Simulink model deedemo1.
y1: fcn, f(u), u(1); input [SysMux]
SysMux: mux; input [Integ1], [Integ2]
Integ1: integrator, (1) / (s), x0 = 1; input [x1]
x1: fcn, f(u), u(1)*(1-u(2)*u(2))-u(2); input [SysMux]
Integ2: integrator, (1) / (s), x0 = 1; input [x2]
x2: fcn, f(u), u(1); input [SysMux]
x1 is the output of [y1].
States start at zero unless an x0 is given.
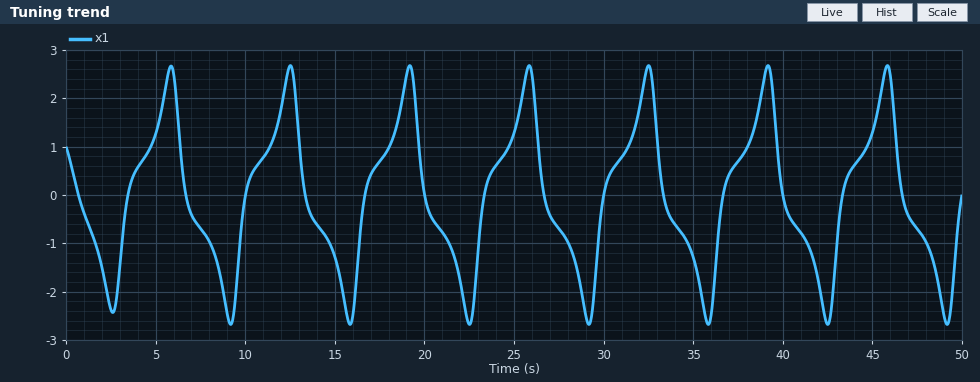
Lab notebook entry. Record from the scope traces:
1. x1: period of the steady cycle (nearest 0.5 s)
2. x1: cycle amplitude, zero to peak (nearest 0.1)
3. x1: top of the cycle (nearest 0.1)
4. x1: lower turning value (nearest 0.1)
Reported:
6.5 s
2.7
2.7
-2.7
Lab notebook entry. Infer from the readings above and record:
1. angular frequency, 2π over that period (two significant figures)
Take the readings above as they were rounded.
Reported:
0.97 rad/s
